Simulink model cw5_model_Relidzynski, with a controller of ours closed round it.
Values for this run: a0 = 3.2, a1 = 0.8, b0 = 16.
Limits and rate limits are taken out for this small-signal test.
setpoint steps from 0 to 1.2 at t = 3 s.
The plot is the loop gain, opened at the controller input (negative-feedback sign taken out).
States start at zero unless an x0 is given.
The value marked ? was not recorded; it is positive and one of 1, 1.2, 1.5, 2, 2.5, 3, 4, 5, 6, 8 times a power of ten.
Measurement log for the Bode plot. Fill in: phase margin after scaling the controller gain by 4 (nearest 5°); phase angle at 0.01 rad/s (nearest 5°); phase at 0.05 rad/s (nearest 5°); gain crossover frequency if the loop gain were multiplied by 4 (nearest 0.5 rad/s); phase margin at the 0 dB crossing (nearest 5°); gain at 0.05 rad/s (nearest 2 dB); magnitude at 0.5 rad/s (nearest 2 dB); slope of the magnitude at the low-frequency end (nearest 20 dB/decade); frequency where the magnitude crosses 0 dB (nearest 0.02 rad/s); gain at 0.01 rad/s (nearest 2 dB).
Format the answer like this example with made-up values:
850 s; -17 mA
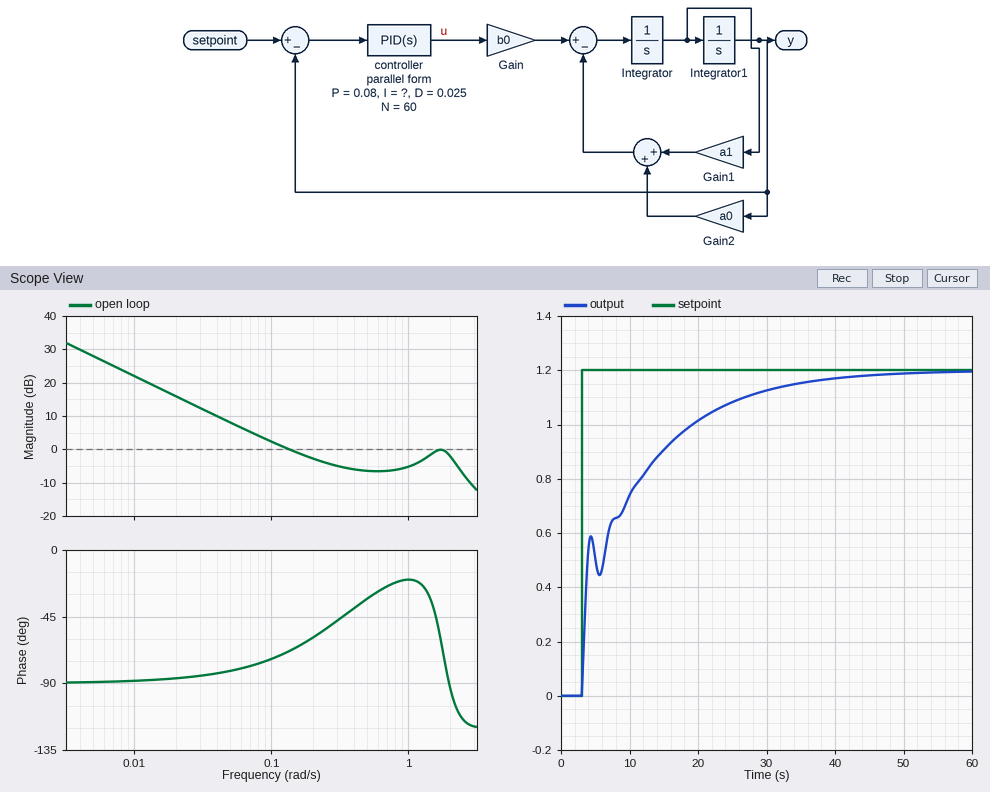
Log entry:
60°; -90°; -80°; 3.0 rad/s; 110°; 8 dB; -6 dB; -20 dB/decade; 0.14 rad/s; 22 dB
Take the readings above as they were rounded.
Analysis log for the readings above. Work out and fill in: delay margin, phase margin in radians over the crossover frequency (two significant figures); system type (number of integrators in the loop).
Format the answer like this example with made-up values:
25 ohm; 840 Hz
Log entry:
14 s; 1
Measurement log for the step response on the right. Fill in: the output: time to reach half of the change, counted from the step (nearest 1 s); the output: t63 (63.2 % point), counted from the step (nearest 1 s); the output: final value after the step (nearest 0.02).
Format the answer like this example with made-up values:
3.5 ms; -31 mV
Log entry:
4 s; 7 s; 1.20
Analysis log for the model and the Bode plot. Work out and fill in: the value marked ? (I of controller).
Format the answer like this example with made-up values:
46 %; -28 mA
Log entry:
0.025
